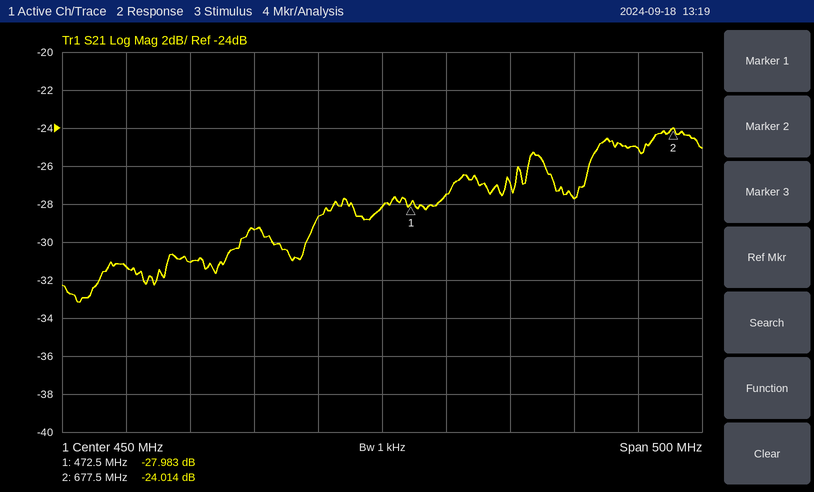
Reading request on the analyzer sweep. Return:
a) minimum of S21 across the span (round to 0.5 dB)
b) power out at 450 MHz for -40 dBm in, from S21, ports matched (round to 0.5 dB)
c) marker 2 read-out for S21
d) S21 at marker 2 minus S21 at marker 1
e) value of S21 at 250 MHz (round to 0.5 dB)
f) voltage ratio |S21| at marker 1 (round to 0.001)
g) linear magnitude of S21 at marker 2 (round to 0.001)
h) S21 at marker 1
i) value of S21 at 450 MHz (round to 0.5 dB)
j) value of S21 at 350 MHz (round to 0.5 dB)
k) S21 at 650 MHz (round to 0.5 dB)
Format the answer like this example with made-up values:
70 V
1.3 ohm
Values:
-33.0 dB
-68.0 dBm
-24.014 dB
3.969 dB
-31.5 dB
0.040
0.063
-27.983 dB
-28.0 dB
-29.5 dB
-25.0 dB
